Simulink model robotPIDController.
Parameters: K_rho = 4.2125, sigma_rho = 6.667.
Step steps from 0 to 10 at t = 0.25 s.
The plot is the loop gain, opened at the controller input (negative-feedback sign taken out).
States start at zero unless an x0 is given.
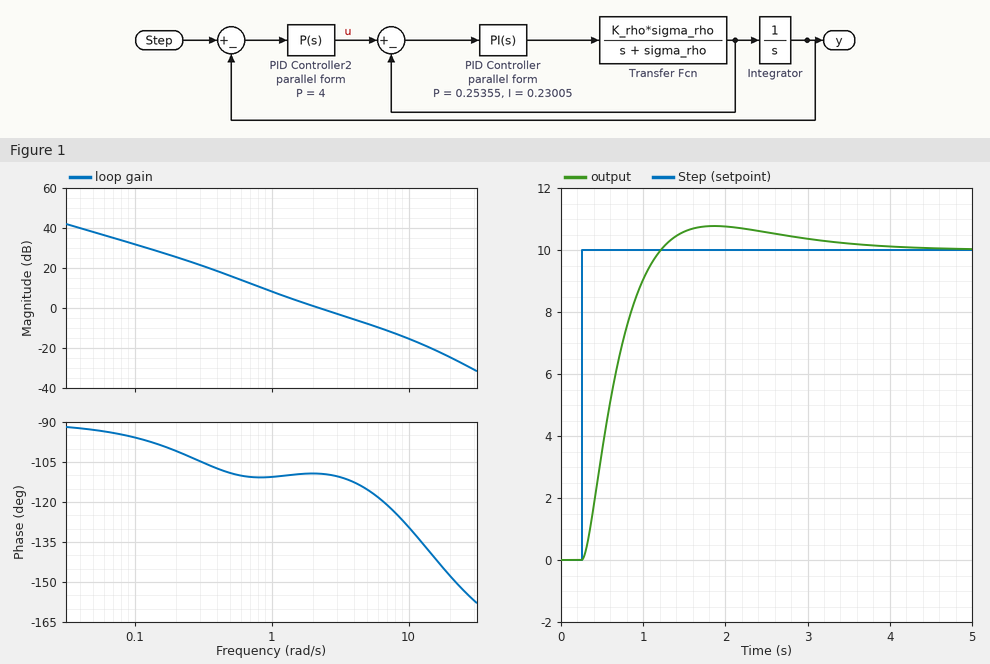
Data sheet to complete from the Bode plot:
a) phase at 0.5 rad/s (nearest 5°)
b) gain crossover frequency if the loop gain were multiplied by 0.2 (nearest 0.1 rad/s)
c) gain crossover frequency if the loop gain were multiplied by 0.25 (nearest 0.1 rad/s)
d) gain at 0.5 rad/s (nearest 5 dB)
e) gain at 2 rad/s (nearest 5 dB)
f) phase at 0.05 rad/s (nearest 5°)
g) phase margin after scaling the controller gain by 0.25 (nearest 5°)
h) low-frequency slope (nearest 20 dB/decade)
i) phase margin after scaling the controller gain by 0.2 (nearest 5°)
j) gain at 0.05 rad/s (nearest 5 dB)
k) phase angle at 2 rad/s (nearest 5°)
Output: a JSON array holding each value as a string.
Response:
["-110°", "0.6 rad/s", "0.7 rad/s", "15 dB", "0 dB", "-95°", "70°", "-20 dB/decade", "70°", "40 dB", "-110°"]
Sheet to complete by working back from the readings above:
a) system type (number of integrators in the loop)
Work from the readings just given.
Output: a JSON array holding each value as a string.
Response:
["1"]
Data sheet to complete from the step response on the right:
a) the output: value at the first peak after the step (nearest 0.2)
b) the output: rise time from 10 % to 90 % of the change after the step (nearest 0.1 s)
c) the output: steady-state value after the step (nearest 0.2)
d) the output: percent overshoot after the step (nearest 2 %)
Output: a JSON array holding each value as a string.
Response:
["10.8", "0.6 s", "10.0", "8 %"]
